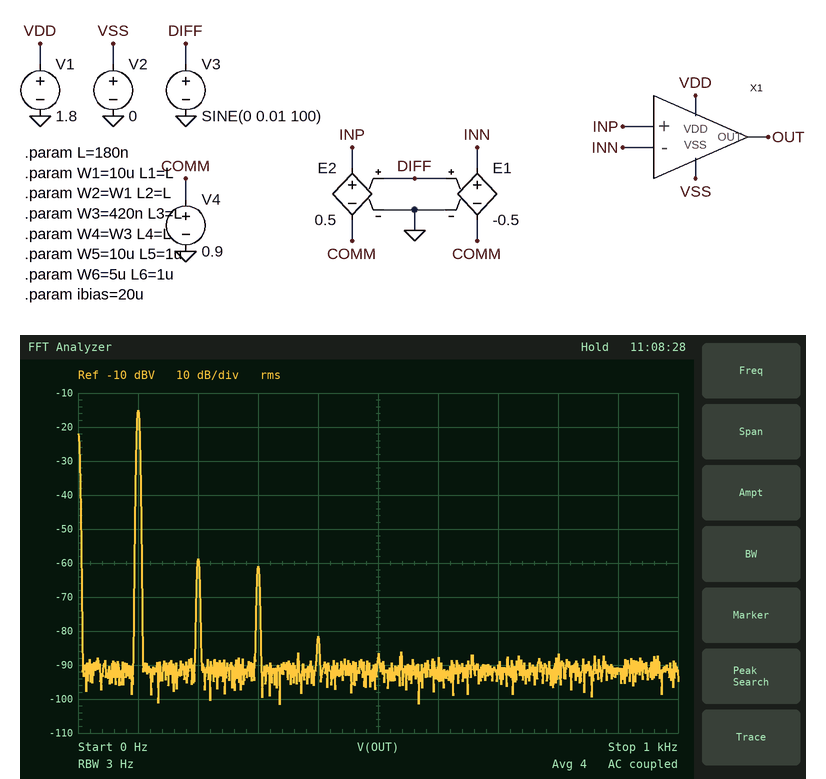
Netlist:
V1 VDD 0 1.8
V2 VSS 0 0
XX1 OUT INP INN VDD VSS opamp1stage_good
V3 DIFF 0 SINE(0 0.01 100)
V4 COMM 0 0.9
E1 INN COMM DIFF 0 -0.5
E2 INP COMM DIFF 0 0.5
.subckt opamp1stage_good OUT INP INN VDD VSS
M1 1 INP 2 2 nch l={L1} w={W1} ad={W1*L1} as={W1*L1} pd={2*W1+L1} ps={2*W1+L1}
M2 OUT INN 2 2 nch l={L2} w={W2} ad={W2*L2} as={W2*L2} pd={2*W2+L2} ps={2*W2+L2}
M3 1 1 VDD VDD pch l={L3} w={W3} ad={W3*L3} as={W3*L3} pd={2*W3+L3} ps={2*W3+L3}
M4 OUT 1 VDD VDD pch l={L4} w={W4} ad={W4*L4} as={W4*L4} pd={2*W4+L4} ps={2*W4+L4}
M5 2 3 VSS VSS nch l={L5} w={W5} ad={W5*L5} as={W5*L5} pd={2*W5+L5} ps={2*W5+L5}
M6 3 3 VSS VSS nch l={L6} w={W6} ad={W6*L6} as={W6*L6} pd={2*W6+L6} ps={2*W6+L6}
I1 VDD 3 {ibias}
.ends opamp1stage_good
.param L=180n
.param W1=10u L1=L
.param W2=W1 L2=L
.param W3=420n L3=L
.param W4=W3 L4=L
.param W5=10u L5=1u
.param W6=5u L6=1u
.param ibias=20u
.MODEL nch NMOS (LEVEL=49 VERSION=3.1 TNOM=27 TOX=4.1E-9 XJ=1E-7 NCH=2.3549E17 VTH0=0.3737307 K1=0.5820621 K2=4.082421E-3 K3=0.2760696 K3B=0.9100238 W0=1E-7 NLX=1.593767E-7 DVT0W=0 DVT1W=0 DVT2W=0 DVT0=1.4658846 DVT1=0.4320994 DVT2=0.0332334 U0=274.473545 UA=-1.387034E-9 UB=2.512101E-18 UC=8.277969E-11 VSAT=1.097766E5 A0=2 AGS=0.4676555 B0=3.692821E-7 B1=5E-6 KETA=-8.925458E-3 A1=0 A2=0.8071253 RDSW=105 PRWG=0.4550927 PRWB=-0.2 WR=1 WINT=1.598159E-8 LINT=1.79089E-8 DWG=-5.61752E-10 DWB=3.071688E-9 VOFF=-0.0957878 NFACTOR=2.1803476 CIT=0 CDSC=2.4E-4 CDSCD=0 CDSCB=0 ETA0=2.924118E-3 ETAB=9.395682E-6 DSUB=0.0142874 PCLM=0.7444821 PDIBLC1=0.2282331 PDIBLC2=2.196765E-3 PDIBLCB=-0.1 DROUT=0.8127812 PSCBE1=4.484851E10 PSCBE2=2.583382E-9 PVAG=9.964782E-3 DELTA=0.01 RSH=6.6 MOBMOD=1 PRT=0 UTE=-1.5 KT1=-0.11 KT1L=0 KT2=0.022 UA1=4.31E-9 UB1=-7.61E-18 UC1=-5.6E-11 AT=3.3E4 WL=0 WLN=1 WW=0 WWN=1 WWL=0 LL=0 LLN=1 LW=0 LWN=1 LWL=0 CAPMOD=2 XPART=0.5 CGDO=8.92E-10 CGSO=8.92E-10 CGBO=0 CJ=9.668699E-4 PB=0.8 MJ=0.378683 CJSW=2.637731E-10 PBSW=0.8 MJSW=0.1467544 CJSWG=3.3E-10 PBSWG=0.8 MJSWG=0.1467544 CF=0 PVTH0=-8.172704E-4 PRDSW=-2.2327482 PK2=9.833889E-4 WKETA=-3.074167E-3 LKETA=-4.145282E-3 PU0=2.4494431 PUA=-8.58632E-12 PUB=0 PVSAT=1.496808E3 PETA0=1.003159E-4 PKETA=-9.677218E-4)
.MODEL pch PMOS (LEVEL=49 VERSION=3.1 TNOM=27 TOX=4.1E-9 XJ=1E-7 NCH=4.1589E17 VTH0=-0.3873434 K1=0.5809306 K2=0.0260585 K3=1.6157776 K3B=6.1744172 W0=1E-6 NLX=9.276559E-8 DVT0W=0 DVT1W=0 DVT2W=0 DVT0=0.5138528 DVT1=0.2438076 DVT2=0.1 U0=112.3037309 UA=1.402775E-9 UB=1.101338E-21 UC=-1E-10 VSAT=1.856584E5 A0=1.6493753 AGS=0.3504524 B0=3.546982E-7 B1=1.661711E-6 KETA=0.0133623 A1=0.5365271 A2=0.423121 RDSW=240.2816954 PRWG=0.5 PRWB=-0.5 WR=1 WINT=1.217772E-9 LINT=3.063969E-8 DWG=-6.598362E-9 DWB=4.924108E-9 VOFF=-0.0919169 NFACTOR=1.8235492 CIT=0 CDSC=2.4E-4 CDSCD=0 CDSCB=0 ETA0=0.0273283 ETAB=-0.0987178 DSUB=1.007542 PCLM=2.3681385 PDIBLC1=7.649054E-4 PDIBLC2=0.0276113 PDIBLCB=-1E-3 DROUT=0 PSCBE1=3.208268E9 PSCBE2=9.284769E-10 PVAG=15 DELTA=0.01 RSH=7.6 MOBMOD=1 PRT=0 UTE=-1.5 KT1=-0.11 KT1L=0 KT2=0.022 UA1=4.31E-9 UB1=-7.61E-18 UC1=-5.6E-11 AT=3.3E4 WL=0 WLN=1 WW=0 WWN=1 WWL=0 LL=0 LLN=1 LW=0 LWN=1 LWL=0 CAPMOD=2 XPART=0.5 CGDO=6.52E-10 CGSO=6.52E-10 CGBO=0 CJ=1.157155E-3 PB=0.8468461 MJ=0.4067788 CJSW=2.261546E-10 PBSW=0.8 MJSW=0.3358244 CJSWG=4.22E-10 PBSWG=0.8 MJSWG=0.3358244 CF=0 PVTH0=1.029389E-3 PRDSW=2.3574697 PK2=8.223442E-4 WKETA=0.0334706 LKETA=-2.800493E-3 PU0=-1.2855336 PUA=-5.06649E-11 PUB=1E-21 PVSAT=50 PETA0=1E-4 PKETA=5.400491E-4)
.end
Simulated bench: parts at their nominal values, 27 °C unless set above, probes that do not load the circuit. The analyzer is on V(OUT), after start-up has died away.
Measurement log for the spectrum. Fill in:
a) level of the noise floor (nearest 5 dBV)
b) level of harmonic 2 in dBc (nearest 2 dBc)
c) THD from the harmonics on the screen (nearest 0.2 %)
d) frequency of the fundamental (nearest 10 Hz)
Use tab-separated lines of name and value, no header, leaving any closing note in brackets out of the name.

level of the noise floor	-90 dBV
level of harmonic 2 in dBc	-44 dBc
THD from the harmonics on the screen	0.8 %
frequency of the fundamental	100 Hz
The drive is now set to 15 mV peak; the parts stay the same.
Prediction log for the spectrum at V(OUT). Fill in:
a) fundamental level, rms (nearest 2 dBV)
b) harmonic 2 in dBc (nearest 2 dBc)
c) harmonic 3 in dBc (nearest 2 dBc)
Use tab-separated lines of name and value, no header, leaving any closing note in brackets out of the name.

fundamental level, rms	-12 dBV
harmonic 2 in dBc	-36 dBc
harmonic 3 in dBc	-36 dBc
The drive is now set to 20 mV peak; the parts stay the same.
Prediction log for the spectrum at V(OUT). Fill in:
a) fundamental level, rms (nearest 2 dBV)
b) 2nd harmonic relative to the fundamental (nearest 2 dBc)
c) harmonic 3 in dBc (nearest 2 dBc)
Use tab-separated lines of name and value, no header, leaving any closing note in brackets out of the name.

fundamental level, rms	-10 dBV
2nd harmonic relative to the fundamental	-28 dBc
harmonic 3 in dBc	-28 dBc
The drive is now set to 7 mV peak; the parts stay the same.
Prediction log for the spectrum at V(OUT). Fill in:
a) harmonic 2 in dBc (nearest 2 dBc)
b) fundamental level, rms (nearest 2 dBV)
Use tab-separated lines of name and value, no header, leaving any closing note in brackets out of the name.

harmonic 2 in dBc	-48 dBc
fundamental level, rms	-18 dBV
